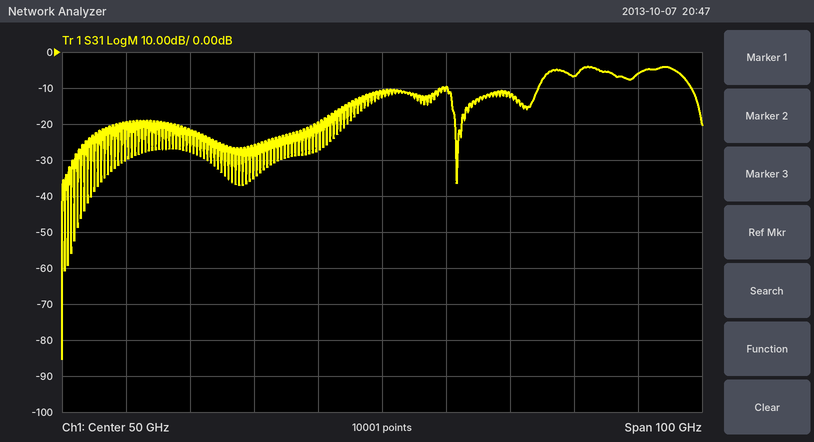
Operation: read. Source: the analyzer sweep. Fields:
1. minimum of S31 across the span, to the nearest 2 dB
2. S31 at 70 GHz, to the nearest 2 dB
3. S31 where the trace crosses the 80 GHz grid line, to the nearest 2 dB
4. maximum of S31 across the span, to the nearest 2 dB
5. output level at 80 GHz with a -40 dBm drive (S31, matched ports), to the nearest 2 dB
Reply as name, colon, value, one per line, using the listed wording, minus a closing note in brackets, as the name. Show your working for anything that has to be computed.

minimum of S31 across the span, to the nearest 2 dB: -86 dB
S31 at 70 GHz, to the nearest 2 dB: -12 dB
S31 where the trace crosses the 80 GHz grid line, to the nearest 2 dB: -6 dB
maximum of S31 across the span, to the nearest 2 dB: -4 dB
output level at 80 GHz with a -40 dBm drive (S31, matched ports), to the nearest 2 dB: -40 dBm + (-6 dB) = -46 dBm
